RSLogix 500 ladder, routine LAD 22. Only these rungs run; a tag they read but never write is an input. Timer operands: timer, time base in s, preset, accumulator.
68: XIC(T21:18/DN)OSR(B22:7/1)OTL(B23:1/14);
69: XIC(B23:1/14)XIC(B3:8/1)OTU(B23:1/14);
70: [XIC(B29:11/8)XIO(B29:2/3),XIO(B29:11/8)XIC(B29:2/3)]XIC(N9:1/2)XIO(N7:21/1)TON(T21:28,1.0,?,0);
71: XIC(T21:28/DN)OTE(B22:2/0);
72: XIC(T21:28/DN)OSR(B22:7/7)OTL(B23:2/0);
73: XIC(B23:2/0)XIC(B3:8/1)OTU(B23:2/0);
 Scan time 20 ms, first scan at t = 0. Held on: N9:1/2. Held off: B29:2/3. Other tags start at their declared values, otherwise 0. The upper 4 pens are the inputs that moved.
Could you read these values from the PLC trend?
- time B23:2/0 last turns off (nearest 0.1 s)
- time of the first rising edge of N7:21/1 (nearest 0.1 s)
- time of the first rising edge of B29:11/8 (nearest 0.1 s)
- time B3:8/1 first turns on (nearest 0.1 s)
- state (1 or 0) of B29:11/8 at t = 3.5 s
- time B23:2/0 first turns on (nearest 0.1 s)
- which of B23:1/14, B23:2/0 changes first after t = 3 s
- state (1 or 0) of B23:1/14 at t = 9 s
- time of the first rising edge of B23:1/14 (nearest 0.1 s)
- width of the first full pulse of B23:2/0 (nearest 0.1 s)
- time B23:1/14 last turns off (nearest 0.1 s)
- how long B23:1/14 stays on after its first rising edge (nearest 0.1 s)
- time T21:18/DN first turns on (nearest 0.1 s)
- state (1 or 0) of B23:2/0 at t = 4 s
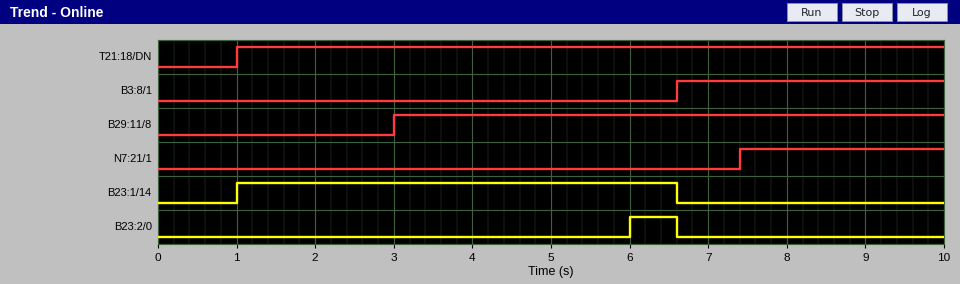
6.6 s
7.4 s
3.0 s
6.6 s
1
6.0 s
B23:2/0
0
1.0 s
0.6 s
6.6 s
5.6 s
1.0 s
0
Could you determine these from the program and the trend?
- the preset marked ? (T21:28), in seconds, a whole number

3 s
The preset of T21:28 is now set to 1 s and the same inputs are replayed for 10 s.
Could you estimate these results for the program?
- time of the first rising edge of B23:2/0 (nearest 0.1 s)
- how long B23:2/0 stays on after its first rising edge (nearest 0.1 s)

4.0 s
2.6 s
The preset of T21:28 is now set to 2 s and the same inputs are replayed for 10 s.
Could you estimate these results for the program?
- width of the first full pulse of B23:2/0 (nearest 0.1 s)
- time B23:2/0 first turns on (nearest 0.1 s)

1.6 s
5.0 s
